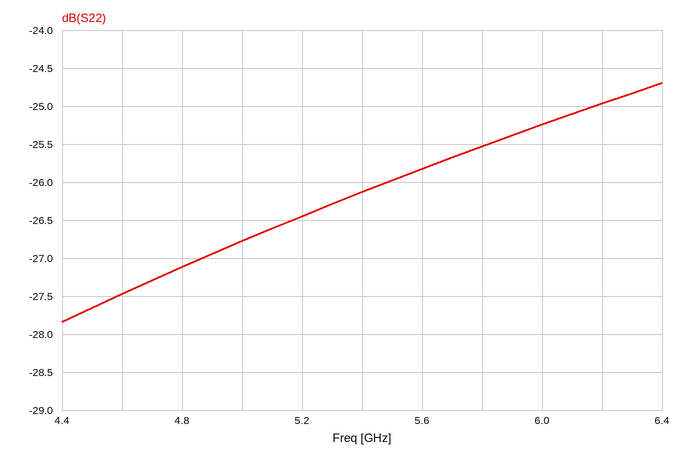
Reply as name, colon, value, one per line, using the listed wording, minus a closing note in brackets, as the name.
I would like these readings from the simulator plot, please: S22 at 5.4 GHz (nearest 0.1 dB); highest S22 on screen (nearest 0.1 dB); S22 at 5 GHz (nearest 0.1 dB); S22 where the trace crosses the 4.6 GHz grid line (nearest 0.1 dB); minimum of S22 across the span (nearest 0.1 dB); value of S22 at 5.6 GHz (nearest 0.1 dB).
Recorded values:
S22 at 5.4 GHz: -26.1 dB
highest S22 on screen: -24.7 dB
S22 at 5 GHz: -26.8 dB
S22 where the trace crosses the 4.6 GHz grid line: -27.5 dB
minimum of S22 across the span: -27.8 dB
value of S22 at 5.6 GHz: -25.8 dB
